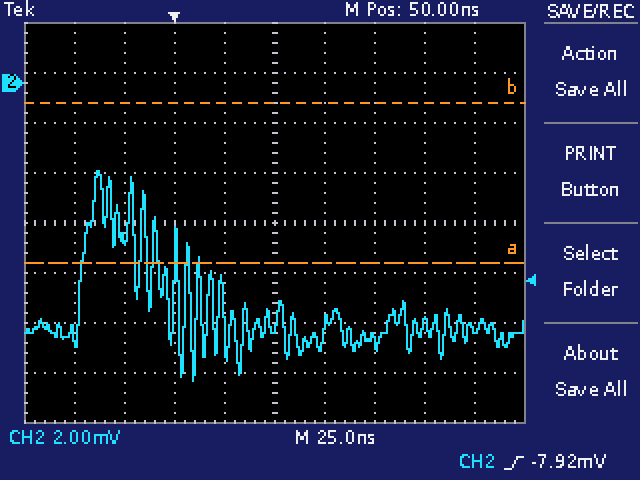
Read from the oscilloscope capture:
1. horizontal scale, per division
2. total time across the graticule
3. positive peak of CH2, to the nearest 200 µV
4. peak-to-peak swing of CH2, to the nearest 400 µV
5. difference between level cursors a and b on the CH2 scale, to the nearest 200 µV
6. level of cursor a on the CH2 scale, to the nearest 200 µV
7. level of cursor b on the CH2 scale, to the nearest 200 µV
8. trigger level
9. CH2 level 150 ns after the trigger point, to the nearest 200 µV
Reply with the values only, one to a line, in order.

25 ns
250 ns
-3.6 mV
8.4 mV
6.4 mV
-7.2 mV
-800 µV
-7.92 mV
-9.8 mV
